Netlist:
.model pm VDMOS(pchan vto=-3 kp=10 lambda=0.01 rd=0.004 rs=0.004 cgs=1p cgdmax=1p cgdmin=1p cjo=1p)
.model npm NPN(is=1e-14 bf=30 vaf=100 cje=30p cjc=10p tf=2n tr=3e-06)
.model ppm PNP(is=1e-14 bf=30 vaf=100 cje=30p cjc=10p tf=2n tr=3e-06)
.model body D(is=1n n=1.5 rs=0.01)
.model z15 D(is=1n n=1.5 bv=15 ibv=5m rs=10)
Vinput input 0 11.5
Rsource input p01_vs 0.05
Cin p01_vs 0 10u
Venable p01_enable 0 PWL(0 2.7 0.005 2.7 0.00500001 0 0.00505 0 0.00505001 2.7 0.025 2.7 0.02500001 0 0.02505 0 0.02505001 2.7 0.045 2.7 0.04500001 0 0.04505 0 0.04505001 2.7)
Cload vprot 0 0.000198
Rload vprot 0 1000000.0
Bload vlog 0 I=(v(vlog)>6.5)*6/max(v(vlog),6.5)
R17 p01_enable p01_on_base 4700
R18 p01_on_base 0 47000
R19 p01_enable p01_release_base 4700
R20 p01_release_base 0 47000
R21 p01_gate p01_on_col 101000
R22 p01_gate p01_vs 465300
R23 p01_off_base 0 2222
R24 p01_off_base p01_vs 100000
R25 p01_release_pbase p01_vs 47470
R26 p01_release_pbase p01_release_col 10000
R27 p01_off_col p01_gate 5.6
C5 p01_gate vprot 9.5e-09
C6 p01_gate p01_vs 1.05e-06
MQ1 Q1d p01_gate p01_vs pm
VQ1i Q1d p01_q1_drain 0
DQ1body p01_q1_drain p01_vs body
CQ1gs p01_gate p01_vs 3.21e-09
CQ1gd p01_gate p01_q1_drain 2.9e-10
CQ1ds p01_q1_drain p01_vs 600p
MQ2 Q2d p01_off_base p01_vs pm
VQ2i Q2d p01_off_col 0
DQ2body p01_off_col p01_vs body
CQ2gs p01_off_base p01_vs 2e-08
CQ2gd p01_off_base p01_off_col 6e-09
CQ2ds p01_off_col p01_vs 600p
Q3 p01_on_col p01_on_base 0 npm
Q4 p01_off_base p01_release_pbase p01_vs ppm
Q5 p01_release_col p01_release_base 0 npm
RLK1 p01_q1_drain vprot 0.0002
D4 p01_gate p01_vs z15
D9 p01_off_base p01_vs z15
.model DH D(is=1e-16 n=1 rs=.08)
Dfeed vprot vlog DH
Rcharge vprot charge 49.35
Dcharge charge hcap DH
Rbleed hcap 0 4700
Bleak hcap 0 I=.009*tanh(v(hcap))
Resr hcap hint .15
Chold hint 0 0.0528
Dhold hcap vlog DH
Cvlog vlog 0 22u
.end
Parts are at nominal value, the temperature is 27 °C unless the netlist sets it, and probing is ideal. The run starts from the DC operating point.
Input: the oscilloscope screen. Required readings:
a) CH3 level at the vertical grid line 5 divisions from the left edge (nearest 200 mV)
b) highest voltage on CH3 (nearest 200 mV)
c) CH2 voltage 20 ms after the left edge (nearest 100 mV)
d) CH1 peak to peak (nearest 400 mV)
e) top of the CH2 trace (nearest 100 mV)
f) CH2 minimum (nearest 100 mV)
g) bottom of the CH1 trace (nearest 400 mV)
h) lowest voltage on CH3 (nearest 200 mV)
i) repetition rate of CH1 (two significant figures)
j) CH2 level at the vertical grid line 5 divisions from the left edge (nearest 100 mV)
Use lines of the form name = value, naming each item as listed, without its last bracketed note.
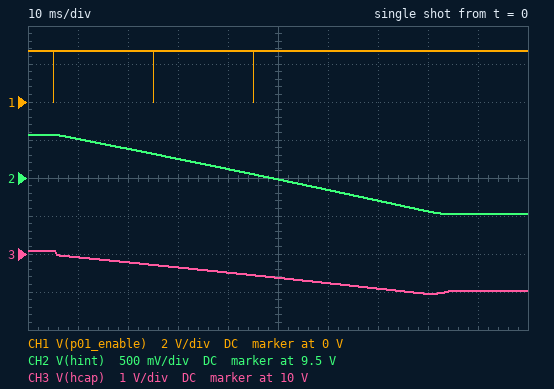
CH3 level at the vertical grid line 5 divisions from the left edge = 9.4 V
highest voltage on CH3 = 10.0 V
CH2 voltage 20 ms after the left edge = 9.9 V
CH1 peak to peak = 2.8 V
top of the CH2 trace = 10.1 V
CH2 minimum = 9.0 V
bottom of the CH1 trace = 0 V
lowest voltage on CH3 = 9.0 V
repetition rate of CH1 = 50 Hz
CH2 level at the vertical grid line 5 divisions from the left edge = 9.5 V
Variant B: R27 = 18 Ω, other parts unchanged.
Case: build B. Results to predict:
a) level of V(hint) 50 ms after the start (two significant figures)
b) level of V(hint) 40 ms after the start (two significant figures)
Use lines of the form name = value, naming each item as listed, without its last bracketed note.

level of V(hint) 50 ms after the start = 9.8 V
level of V(hint) 40 ms after the start = 9.9 V
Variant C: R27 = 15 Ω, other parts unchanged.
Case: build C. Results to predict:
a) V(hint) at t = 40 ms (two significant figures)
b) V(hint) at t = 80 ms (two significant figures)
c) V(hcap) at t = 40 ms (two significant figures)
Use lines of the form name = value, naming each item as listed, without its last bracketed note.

V(hint) at t = 40 ms = 9.9 V
V(hint) at t = 80 ms = 9.4 V
V(hcap) at t = 40 ms = 9.8 V
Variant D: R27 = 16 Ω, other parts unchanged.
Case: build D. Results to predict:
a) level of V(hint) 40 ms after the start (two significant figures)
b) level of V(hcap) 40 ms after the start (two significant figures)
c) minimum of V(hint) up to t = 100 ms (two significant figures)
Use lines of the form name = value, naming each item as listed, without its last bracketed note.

level of V(hint) 40 ms after the start = 9.9 V
level of V(hcap) 40 ms after the start = 9.8 V
minimum of V(hint) up to t = 100 ms = 9.4 V
